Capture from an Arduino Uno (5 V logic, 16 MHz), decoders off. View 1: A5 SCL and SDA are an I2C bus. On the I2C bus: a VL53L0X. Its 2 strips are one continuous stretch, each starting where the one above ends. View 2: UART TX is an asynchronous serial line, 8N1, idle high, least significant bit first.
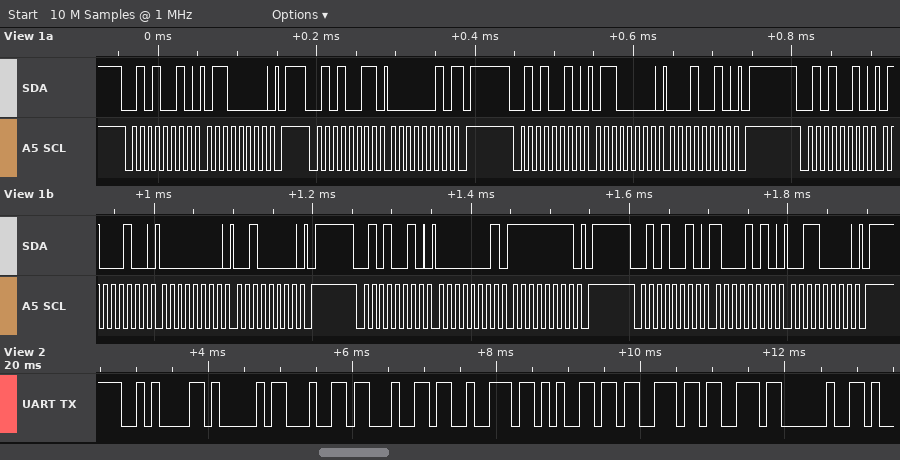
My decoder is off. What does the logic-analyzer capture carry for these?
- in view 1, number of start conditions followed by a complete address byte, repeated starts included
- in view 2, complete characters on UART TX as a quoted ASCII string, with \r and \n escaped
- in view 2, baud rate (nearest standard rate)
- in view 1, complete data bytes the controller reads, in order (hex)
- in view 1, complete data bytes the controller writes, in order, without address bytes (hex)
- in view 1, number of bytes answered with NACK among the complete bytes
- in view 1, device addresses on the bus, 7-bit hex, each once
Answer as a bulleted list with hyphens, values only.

- 6
- "\nAddress "
- 9600 baud
- 02
- 60 60 12 44 00 20 01 FF 8A 30
- 1
- 0x29
